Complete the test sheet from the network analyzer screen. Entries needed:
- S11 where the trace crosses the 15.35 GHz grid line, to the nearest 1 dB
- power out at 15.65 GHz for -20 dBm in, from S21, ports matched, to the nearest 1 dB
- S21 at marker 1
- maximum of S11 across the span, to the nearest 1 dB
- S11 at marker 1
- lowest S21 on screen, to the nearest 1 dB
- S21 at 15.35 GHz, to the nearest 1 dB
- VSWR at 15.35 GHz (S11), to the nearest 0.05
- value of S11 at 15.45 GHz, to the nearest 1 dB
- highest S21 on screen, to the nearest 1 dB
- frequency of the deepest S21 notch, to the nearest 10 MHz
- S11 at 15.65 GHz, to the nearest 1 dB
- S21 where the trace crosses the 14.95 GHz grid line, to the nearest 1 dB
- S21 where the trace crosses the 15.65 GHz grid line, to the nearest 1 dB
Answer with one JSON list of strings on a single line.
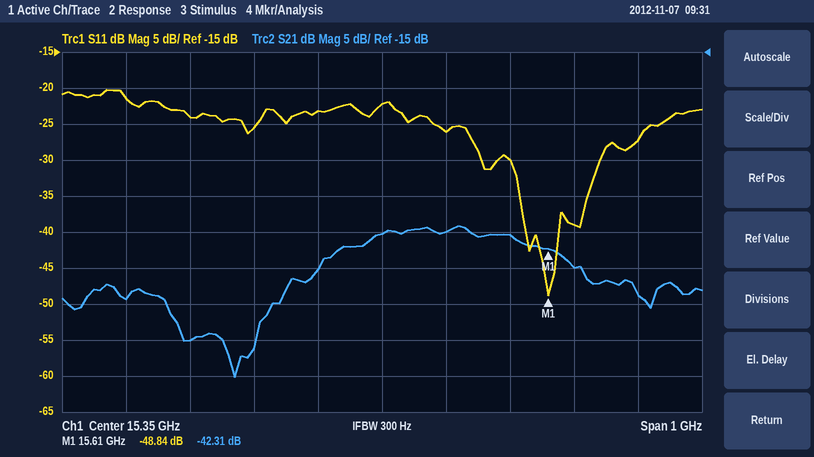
["-22 dB", "-65 dBm", "-42.31 dB", "-20 dB", "-48.84 dB", "-60 dB", "-40 dB", "1.15", "-26 dB", "-39 dB", "15.12 GHz", "-39 dB", "-49 dB", "-45 dB"]
